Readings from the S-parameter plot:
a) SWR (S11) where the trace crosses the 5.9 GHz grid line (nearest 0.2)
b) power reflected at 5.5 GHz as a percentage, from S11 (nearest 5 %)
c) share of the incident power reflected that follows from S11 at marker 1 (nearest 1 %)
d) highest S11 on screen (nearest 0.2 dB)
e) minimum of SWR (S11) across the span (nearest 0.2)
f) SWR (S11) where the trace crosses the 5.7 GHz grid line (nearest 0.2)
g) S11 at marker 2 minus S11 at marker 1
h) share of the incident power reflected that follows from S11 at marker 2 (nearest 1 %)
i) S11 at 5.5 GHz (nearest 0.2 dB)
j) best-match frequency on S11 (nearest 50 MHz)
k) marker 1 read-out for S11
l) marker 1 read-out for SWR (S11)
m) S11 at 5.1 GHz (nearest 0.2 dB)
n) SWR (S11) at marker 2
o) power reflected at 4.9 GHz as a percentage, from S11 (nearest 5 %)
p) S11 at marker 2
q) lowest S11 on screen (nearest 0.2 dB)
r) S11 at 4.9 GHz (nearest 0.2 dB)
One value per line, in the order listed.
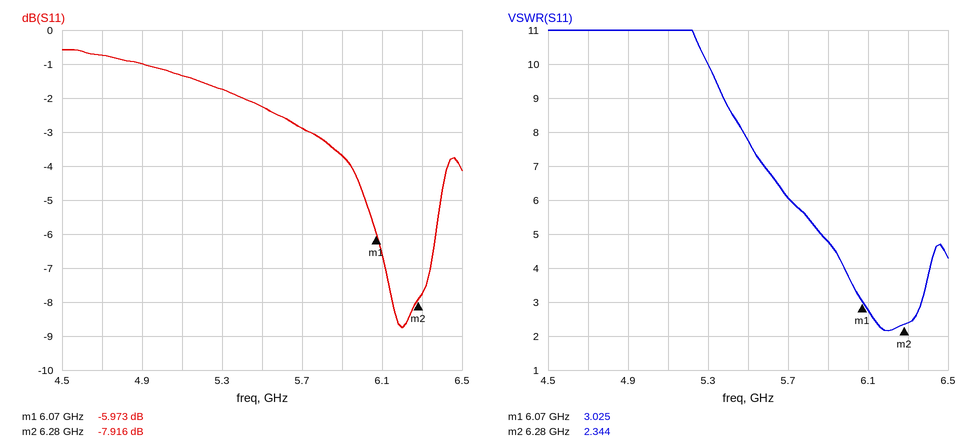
4.8
60 %
25 %
-0.6 dB
2.2
6.0
-1.943 dB
16 %
-2.2 dB
6.20 GHz
-5.973 dB
3.025
-1.4 dB
2.344
80 %
-7.916 dB
-8.8 dB
-1.0 dB
